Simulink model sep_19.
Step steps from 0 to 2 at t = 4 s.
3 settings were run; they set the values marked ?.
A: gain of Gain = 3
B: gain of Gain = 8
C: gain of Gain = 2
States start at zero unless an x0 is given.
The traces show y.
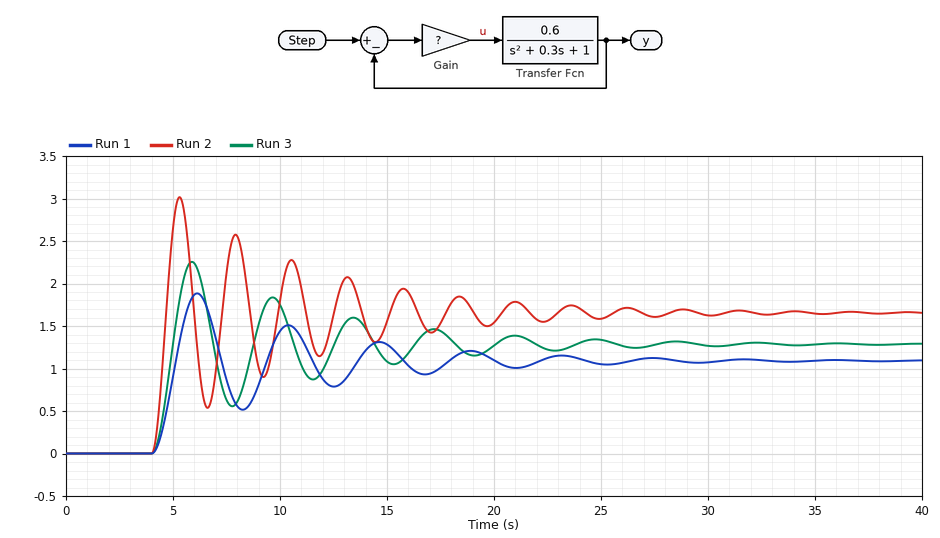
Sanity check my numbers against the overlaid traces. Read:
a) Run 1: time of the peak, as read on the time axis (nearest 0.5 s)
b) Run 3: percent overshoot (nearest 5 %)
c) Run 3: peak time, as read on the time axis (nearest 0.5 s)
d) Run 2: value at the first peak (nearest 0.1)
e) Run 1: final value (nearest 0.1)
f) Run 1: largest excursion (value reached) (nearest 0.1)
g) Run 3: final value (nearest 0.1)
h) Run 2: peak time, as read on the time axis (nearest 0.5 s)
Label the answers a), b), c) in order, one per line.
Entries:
a) 6.0 s
b) 75 %
c) 6.0 s
d) 3.0
e) 1.1
f) 1.9
g) 1.3
h) 5.5 s
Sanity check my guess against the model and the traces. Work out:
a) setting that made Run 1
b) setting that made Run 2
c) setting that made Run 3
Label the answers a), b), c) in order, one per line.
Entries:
a) C
b) B
c) A
